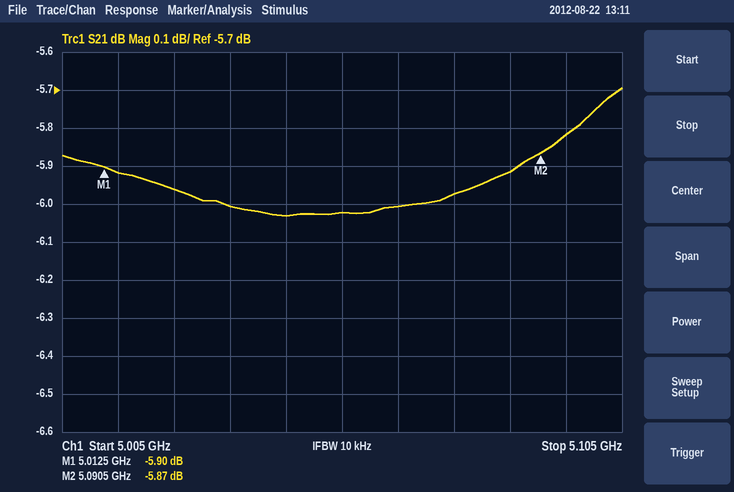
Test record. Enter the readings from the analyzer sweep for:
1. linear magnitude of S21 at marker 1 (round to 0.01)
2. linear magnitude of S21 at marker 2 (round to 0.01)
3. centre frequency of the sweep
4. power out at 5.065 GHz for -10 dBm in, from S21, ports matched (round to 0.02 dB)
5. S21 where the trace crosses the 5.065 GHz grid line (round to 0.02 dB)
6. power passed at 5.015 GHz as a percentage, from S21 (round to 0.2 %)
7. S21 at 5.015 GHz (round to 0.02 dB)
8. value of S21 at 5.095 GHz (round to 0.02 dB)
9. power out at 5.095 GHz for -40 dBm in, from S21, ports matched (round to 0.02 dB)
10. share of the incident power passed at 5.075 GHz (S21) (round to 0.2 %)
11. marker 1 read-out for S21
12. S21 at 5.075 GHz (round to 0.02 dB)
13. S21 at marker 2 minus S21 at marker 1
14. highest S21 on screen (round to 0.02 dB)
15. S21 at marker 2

0.51
0.51
5.055 GHz
-16.00 dBm
-6.00 dB
25.6 %
-5.92 dB
-5.82 dB
-45.82 dBm
25.2 %
-5.90 dB
-5.98 dB
0.03 dB
-5.70 dB
-5.87 dB
